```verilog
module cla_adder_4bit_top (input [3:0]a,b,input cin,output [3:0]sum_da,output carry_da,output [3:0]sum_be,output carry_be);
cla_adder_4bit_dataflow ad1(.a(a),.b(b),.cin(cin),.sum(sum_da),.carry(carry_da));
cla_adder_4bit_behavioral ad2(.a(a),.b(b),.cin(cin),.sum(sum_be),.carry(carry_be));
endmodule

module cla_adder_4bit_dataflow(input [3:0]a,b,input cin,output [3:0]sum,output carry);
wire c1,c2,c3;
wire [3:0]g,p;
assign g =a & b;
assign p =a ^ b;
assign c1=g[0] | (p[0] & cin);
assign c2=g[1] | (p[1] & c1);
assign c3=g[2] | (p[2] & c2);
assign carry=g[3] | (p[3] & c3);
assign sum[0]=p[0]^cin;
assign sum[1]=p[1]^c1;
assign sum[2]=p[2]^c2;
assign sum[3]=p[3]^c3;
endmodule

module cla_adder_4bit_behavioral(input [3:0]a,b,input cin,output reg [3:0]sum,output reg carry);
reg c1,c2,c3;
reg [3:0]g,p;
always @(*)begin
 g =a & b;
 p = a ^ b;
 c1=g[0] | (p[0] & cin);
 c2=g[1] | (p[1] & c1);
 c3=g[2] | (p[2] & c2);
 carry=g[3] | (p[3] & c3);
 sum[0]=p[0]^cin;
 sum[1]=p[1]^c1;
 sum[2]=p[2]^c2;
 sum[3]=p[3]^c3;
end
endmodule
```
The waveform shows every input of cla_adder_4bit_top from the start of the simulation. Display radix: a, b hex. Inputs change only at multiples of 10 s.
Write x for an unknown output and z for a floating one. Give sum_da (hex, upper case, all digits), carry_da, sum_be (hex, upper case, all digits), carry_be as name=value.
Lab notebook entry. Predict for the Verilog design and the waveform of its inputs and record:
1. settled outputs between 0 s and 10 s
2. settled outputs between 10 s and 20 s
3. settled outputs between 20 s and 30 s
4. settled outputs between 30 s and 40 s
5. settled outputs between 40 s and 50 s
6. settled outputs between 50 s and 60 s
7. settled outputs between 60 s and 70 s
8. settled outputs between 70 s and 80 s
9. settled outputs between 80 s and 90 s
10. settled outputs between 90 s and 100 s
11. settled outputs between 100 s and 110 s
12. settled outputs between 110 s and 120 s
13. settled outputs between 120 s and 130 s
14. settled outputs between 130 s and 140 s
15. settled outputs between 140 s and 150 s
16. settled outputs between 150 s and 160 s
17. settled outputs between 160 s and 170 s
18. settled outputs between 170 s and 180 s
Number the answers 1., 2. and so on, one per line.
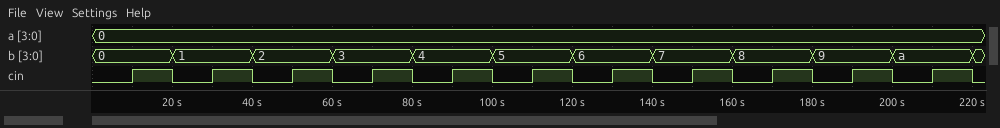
1. sum_da=0, carry_da=0, sum_be=0, carry_be=0
2. sum_da=1, carry_da=0, sum_be=1, carry_be=0
3. sum_da=1, carry_da=0, sum_be=1, carry_be=0
4. sum_da=2, carry_da=0, sum_be=2, carry_be=0
5. sum_da=2, carry_da=0, sum_be=2, carry_be=0
6. sum_da=3, carry_da=0, sum_be=3, carry_be=0
7. sum_da=3, carry_da=0, sum_be=3, carry_be=0
8. sum_da=4, carry_da=0, sum_be=4, carry_be=0
9. sum_da=4, carry_da=0, sum_be=4, carry_be=0
10. sum_da=5, carry_da=0, sum_be=5, carry_be=0
11. sum_da=5, carry_da=0, sum_be=5, carry_be=0
12. sum_da=6, carry_da=0, sum_be=6, carry_be=0
13. sum_da=6, carry_da=0, sum_be=6, carry_be=0
14. sum_da=7, carry_da=0, sum_be=7, carry_be=0
15. sum_da=7, carry_da=0, sum_be=7, carry_be=0
16. sum_da=8, carry_da=0, sum_be=8, carry_be=0
17. sum_da=8, carry_da=0, sum_be=8, carry_be=0
18. sum_da=9, carry_da=0, sum_be=9, carry_be=0
